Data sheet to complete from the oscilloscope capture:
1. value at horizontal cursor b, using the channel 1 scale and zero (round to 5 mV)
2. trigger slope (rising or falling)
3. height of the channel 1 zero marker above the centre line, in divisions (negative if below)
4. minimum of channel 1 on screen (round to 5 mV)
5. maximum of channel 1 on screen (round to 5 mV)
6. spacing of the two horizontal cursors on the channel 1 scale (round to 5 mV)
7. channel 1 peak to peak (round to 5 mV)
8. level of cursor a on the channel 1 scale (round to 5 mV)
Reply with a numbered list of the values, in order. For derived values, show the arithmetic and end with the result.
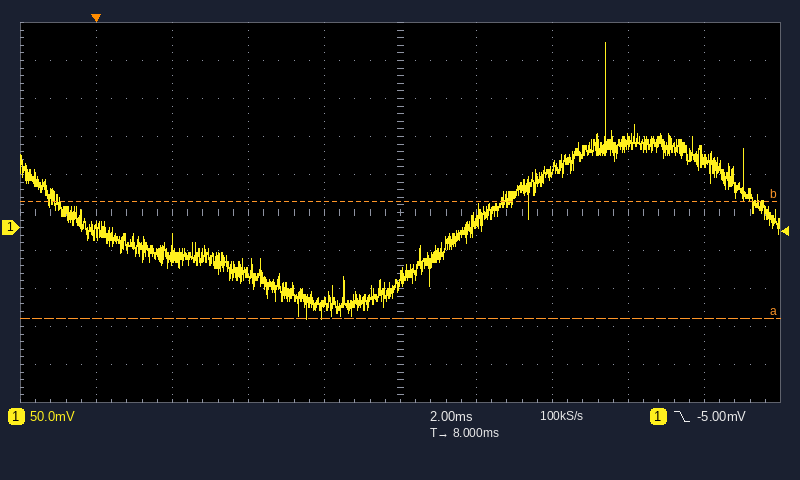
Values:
1. 35 mV
2. falling
3. -0.4 div
4. -120 mV
5. 245 mV
6. 155 mV
7. 245 mV − (-120 mV) = 365 mV
8. -120 mV
